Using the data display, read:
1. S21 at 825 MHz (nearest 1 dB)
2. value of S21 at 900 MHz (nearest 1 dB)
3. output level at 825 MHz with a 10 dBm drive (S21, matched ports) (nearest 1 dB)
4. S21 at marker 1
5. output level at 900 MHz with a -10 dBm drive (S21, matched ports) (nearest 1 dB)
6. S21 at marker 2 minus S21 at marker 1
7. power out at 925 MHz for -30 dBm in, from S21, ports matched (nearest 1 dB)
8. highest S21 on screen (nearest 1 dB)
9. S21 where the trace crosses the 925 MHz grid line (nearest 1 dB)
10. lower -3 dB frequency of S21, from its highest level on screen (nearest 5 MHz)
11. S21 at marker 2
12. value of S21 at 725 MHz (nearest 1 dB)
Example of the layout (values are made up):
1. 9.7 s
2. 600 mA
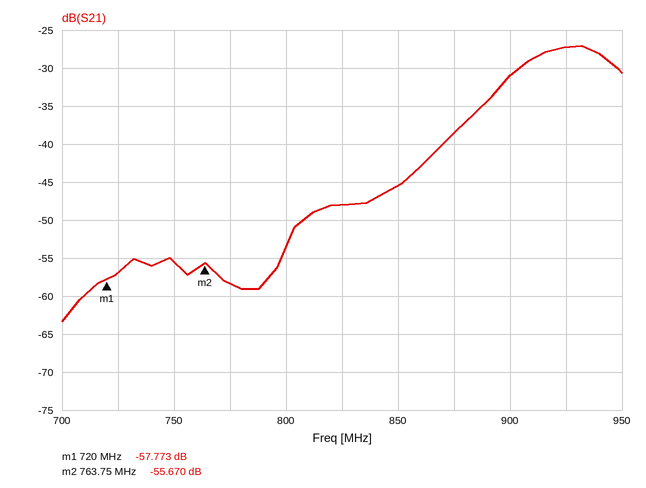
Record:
1. -48 dB
2. -31 dB
3. -38 dBm
4. -57.773 dB
5. -41 dBm
6. 2.103 dB
7. -57 dBm
8. -27 dB
9. -27 dB
10. 905 MHz
11. -55.670 dB
12. -57 dB
